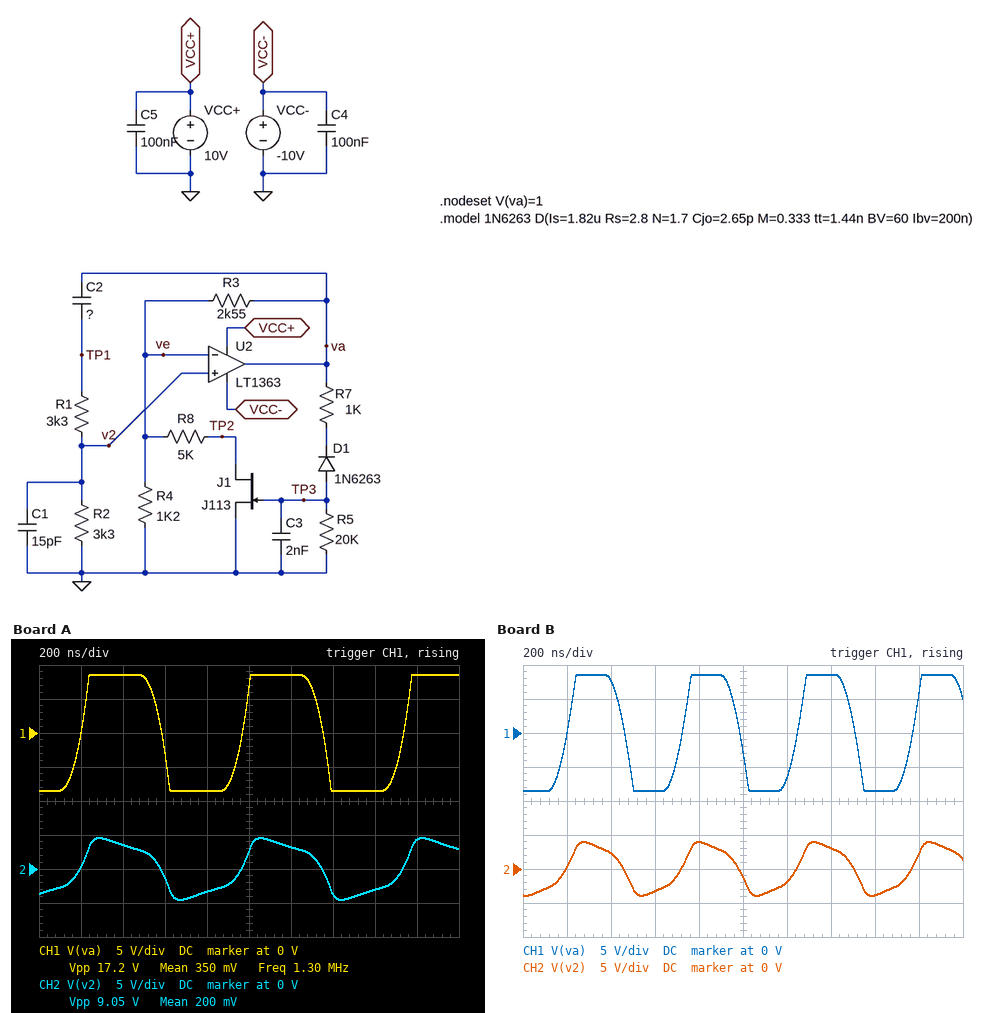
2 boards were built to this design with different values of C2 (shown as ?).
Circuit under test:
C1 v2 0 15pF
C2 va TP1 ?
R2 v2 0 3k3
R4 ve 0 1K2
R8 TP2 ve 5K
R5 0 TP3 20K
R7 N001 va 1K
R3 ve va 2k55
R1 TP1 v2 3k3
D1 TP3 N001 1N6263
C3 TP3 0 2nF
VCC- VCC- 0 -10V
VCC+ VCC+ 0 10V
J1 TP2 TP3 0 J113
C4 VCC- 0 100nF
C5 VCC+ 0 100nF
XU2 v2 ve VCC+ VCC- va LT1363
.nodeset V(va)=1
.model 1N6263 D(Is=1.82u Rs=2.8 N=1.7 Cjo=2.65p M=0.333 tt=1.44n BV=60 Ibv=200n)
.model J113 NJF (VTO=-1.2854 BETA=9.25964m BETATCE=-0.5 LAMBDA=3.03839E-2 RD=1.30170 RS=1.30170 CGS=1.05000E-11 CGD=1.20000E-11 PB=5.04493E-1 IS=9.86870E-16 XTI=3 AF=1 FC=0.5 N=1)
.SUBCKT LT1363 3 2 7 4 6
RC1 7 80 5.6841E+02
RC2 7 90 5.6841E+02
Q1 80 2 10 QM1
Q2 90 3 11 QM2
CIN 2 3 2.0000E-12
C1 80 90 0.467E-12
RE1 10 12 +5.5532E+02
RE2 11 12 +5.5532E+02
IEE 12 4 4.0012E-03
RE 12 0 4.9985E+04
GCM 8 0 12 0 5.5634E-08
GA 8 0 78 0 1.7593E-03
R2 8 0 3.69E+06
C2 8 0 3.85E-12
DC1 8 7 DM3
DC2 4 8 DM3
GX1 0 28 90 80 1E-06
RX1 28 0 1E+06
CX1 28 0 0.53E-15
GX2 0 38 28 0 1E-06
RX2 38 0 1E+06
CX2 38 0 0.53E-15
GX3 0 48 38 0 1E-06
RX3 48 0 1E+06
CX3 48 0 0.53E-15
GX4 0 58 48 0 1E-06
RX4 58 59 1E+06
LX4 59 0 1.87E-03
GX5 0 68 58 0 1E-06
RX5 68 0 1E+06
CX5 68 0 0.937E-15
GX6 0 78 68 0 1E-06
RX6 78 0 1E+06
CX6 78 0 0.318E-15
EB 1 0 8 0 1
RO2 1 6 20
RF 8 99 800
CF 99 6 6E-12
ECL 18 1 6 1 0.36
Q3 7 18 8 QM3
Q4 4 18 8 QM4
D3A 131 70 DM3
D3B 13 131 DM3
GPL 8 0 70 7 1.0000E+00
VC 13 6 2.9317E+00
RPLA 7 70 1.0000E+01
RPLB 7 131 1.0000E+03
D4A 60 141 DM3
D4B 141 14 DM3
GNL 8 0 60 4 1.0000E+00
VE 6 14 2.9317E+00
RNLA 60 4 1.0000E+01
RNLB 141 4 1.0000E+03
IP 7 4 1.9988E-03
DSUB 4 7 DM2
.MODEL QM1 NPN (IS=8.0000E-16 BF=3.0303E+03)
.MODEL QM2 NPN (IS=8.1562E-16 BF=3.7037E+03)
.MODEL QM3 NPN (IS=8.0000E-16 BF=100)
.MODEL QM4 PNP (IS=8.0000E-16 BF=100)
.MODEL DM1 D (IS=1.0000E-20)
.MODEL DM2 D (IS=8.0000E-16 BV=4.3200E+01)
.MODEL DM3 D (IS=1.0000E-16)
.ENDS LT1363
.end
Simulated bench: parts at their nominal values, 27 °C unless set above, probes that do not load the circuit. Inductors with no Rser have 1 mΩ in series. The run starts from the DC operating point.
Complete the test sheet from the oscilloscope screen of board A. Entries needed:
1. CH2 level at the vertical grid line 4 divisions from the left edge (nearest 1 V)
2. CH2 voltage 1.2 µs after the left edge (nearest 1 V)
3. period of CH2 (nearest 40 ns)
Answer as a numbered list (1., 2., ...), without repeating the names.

1. -3 V
2. 3 V
3. 760 ns
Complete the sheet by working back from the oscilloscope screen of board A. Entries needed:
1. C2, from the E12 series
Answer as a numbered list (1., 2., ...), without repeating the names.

1. 47 pF
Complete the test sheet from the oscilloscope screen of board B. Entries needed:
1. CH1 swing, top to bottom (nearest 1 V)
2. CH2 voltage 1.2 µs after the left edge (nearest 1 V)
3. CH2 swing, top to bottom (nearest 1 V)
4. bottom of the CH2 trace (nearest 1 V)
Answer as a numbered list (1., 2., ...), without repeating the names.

1. 17 V
2. -2 V
3. 8 V
4. -4 V
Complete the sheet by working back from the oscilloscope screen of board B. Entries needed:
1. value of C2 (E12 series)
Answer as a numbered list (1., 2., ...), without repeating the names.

1. 27 pF
